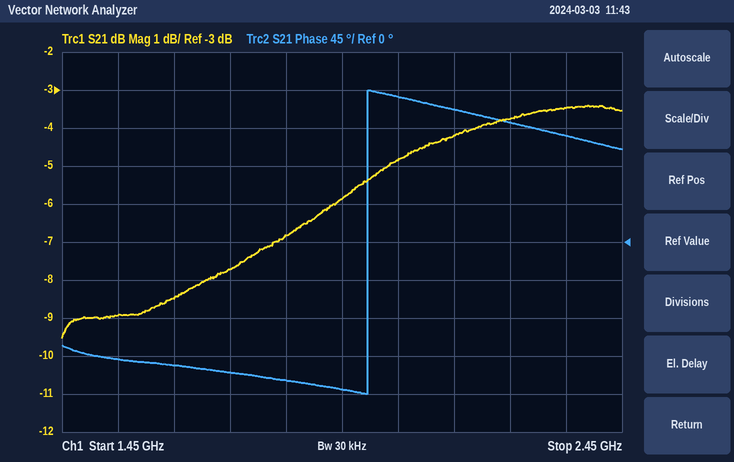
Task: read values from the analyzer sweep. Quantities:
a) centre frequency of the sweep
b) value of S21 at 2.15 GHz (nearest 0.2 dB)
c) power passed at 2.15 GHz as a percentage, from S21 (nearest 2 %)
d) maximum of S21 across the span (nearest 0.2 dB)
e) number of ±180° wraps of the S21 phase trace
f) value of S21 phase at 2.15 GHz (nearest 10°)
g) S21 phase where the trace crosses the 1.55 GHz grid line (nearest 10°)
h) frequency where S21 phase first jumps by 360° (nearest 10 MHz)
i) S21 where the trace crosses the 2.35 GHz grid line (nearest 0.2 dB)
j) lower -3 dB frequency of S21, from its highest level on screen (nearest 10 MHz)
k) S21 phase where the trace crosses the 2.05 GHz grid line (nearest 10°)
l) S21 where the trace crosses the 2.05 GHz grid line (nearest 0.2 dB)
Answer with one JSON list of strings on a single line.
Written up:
["1.95 GHz", "-4.2 dB", "38 %", "-3.4 dB", "1", "160°", "-140°", "2.00 GHz", "-3.4 dB", "1.90 GHz", "170°", "-4.8 dB"]
